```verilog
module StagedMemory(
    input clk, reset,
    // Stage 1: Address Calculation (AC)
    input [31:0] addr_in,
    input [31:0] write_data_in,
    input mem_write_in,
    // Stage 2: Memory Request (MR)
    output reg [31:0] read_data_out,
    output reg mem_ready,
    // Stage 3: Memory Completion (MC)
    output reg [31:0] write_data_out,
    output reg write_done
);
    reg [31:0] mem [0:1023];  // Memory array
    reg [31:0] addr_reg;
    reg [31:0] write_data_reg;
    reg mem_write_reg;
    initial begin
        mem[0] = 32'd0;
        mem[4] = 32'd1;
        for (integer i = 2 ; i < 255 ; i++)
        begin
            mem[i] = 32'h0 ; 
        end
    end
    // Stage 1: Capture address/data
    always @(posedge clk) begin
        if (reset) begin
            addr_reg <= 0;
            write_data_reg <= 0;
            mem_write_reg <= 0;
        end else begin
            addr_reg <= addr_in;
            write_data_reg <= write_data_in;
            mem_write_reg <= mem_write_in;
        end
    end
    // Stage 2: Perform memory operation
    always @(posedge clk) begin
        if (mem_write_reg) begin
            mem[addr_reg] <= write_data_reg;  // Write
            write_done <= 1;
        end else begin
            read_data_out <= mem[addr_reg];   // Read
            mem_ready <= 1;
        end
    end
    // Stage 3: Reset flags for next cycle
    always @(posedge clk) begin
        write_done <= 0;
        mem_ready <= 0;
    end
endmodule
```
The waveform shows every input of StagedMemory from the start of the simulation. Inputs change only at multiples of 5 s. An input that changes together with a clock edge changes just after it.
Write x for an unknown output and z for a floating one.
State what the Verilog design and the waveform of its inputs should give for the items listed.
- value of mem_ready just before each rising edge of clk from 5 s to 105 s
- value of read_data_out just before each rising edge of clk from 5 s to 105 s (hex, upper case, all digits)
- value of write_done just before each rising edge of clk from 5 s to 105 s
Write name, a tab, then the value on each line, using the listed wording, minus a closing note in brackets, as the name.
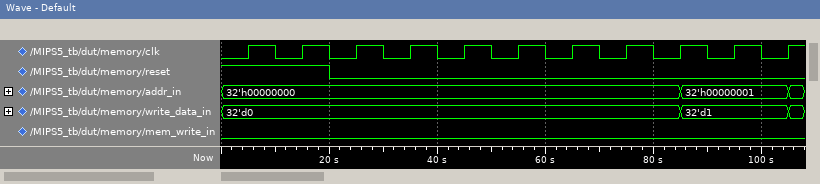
value of mem_ready just before each rising edge of clk from 5 s to 105 s	x 1 0 1 0 1 0 1 0 1 0
value of read_data_out just before each rising edge of clk from 5 s to 105 s	x, x, 00000000, 00000000, 00000000, 00000000, 00000000, 00000000, 00000000, 00000000, 00000000
value of write_done just before each rising edge of clk from 5 s to 105 s	x 0 0 0 0 0 0 0 0 0 0
